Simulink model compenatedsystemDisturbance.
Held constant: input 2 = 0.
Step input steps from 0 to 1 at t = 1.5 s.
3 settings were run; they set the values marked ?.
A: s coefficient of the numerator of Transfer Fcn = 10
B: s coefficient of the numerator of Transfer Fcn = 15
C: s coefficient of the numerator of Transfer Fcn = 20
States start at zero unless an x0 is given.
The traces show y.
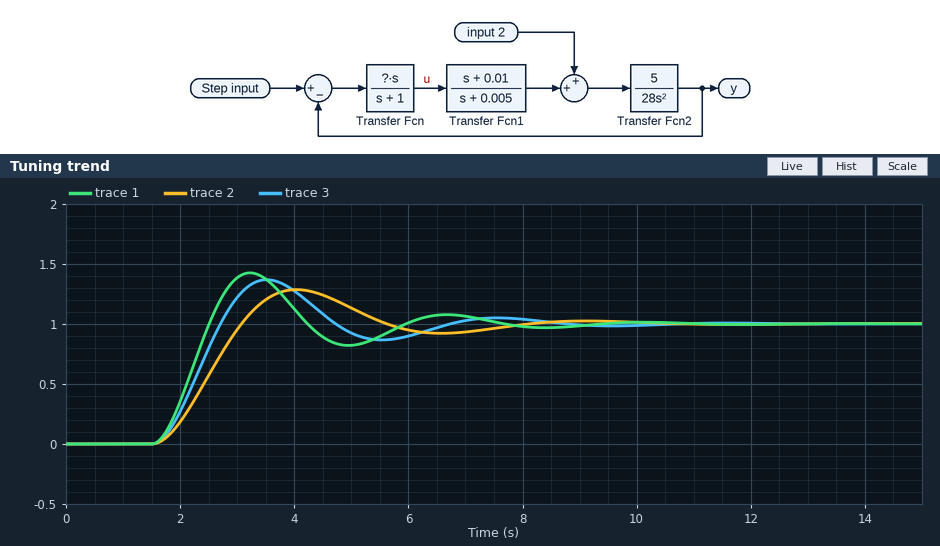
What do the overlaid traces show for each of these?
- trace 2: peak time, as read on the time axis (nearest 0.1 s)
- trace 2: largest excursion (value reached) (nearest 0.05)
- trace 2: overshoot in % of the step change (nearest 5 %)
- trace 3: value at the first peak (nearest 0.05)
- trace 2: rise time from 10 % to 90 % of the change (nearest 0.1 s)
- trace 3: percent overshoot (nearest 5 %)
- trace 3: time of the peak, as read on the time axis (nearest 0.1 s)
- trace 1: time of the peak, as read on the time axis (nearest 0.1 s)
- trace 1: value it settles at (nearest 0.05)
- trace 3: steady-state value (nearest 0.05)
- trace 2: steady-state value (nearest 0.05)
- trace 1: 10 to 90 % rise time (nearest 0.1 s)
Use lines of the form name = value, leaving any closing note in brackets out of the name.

trace 2: peak time, as read on the time axis = 4.0 s
trace 2: largest excursion (value reached) = 1.30
trace 2: overshoot in % of the step change = 30 %
trace 3: value at the first peak = 1.35
trace 2: rise time from 10 % to 90 % of the change = 1.1 s
trace 3: percent overshoot = 35 %
trace 3: time of the peak, as read on the time axis = 3.5 s
trace 1: time of the peak, as read on the time axis = 3.2 s
trace 1: value it settles at = 1.00
trace 3: steady-state value = 1.00
trace 2: steady-state value = 1.00
trace 1: 10 to 90 % rise time = 0.7 s
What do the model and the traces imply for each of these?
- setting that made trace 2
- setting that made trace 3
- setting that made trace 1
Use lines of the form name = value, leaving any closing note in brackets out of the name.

setting that made trace 2 = A
setting that made trace 3 = B
setting that made trace 1 = C
